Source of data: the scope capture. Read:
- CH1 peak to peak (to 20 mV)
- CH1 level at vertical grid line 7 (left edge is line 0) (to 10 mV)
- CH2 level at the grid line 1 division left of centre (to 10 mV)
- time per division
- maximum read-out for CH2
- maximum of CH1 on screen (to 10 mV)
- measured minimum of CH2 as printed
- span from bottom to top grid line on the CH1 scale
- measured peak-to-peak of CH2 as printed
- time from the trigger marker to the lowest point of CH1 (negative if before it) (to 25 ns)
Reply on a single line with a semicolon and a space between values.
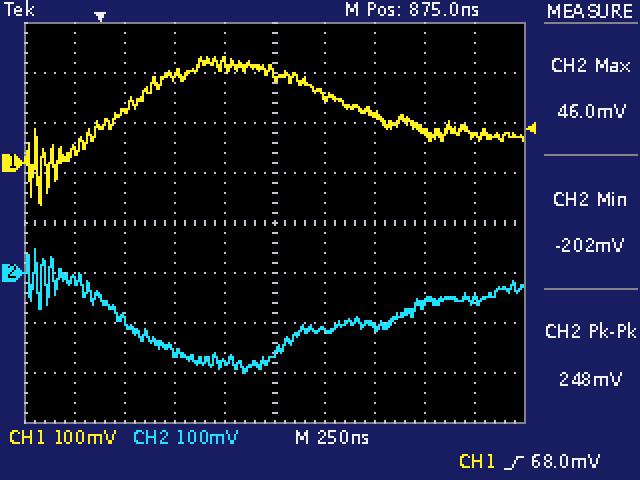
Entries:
300 mV; 100 mV; -180 mV; 250 ns; 46.0 mV; 210 mV; -202 mV; 800 mV; 248 mV; -300 ns
